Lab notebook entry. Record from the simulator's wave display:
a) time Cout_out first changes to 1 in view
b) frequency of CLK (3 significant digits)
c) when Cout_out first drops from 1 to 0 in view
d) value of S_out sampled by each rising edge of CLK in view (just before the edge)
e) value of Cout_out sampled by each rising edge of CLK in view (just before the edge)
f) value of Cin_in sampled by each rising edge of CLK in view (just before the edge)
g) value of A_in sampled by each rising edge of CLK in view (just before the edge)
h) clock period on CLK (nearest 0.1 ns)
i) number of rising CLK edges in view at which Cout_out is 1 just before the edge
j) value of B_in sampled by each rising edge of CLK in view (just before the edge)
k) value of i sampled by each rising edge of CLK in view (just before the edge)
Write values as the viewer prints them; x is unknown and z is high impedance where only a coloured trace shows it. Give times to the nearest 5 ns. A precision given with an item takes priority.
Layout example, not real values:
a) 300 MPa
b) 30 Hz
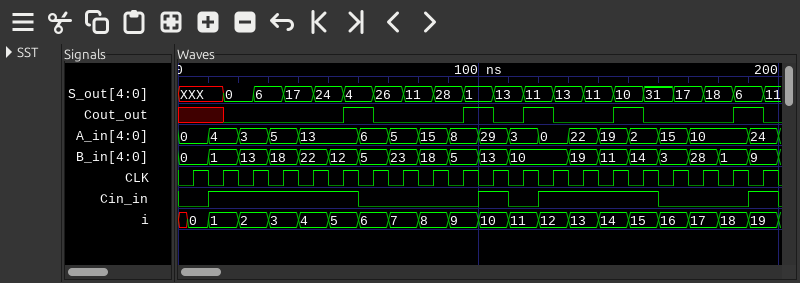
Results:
a) 55 ns
b) 100 MHz
c) 65 ns
d) XXX, XXX, 0, 6, 17, 24, 4, 26, 11, 28, 1, 13, 11, 13, 11, 10, 31, 17, 18, 6
e) x x 0 0 0 0 1 0 0 0 1 0 1 0 0 1 0 0 0 1
f) 0 1 1 1 1 1 0 0 0 0 1 0 1 1 1 1 0 0 0 1
g) 0, 4, 3, 5, 13, 13, 6, 5, 15, 8, 29, 3, 0, 22, 19, 2, 15, 10, 10, 24
h) 10 ns
i) 5
j) 0, 1, 13, 18, 22, 12, 5, 23, 18, 5, 13, 10, 10, 19, 11, 14, 3, 28, 1, 9
k) 0, 1, 2, 3, 4, 5, 6, 7, 8, 9, 10, 11, 12, 13, 14, 15, 16, 17, 18, 19
